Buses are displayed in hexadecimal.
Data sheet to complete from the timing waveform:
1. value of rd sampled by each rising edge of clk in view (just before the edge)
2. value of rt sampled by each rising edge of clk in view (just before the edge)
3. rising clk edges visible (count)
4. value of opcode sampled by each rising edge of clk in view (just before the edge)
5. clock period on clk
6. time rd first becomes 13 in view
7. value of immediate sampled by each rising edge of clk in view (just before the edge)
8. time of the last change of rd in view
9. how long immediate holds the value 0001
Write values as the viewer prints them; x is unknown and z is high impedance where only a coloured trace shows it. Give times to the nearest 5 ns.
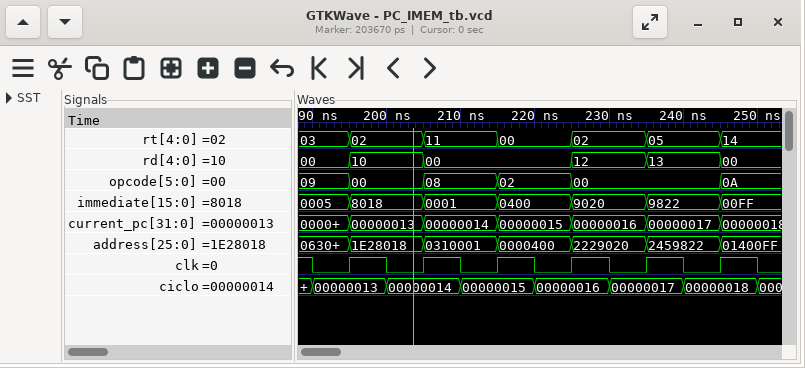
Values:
00, 10, 00, 00, 12, 13
03, 02, 11, 00, 02, 05
6
09, 00, 08, 02, 00, 00
10 ns
235 ns
0005, 8018, 0001, 0400, 9020, 9822
245 ns
10 ns
